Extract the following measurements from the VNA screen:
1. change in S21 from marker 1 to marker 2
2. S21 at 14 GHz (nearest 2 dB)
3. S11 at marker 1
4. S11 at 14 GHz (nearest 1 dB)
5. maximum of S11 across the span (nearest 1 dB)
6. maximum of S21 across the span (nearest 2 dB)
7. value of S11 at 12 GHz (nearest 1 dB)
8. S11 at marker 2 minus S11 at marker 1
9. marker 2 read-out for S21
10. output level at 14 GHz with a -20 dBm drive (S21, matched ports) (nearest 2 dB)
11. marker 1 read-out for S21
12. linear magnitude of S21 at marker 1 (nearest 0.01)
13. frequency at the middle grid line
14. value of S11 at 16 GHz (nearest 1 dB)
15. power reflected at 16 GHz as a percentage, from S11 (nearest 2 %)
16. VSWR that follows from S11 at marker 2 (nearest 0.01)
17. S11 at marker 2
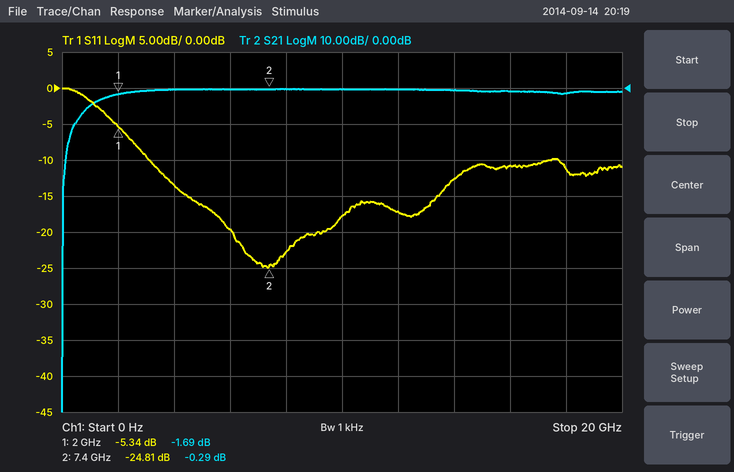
1.40 dB
0 dB
-5.34 dB
-13 dB
0 dB
0 dB
-17 dB
-19.47 dB
-0.29 dB
-20 dBm
-1.69 dB
0.82
10 GHz
-11 dB
8 %
1.12
-24.81 dB
